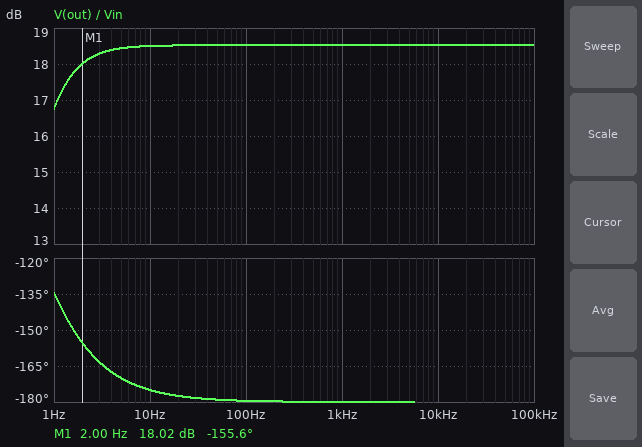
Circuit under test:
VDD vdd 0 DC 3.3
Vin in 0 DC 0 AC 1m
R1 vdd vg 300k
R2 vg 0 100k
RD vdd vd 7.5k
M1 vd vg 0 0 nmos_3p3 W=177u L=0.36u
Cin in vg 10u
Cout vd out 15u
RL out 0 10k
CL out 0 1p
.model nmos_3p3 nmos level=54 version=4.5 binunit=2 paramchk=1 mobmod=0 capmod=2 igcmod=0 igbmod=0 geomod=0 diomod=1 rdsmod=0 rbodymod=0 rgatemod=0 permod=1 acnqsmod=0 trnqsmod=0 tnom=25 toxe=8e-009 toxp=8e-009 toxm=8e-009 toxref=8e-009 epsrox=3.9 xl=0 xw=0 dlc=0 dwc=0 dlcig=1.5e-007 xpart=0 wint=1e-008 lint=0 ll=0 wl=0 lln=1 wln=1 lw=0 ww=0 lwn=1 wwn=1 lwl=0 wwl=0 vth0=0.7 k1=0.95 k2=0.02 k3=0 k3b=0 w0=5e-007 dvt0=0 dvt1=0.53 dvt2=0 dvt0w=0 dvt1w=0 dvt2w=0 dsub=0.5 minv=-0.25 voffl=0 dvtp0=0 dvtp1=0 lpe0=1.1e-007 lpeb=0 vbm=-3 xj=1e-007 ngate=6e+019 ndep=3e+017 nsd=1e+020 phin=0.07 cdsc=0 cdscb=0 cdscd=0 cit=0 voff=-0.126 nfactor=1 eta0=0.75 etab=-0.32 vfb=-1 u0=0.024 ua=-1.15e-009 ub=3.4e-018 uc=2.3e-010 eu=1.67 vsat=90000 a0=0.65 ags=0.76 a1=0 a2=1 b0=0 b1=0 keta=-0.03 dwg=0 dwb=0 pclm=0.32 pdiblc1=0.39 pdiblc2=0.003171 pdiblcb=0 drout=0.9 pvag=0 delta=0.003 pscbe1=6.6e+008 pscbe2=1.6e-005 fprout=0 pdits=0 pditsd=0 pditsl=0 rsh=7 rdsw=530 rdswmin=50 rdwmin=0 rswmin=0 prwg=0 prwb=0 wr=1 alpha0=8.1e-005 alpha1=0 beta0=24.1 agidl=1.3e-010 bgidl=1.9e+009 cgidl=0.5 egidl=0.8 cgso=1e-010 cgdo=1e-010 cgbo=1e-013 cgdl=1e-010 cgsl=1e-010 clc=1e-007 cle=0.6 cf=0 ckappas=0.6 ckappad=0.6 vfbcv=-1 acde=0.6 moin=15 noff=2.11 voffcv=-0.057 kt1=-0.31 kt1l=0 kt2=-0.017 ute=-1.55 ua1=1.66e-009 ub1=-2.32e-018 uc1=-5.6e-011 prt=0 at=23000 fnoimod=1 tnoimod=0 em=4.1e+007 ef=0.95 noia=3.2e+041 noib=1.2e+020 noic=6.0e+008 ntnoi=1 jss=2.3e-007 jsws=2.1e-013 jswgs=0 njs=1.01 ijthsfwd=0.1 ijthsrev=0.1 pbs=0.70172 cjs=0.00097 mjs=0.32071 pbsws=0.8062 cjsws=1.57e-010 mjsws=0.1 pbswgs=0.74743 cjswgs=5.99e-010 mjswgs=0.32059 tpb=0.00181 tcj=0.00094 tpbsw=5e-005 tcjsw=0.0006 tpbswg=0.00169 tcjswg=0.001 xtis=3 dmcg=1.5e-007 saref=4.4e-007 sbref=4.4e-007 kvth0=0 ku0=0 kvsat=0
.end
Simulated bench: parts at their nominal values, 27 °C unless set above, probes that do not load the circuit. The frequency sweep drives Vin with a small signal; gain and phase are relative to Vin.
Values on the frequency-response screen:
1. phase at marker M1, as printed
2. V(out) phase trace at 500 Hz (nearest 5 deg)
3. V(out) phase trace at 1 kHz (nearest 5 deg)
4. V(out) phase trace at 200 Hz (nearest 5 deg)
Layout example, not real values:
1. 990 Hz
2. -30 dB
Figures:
1. -155.6 deg
2. -180 deg
3. -180 deg
4. -180 deg
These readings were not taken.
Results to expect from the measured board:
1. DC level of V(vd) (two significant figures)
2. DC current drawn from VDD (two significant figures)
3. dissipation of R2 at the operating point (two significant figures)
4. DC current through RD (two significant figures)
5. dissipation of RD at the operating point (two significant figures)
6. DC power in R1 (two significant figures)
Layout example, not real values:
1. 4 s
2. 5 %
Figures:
1. 2.2 V
2. 150 µA
3. 6.8 µW
4. 140 µA
5. 150 µW
6. 20 µW
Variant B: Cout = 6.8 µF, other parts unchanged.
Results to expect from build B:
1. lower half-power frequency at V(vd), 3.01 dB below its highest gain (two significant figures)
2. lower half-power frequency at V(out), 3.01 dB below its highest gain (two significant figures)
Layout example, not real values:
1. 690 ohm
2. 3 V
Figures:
1. 180 mHz
2. 1.5 Hz
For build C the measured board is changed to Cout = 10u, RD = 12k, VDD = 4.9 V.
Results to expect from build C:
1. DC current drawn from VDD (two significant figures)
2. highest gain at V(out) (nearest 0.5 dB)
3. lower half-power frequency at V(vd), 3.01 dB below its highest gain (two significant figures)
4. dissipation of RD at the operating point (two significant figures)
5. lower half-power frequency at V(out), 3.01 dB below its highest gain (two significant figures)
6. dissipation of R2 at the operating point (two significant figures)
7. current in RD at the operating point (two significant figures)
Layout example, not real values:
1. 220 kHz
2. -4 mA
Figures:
1. 420 µA
2. -25.0 dB
3. 210 mHz
4. 2.0 mW
5. 1.6 Hz
6. 15 µW
7. 410 µA
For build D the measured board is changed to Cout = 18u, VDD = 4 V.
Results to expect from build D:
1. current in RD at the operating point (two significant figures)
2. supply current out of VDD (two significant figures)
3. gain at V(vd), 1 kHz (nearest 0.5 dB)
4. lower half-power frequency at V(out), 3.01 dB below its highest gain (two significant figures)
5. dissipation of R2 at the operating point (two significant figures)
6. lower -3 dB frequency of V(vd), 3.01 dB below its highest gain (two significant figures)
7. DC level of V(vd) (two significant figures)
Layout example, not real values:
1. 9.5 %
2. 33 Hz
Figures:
1. 520 µA
2. 530 µA
3. -3.5 dB
4. 910 mHz
5. 10 µW
6. 200 mHz
7. 78 mV
